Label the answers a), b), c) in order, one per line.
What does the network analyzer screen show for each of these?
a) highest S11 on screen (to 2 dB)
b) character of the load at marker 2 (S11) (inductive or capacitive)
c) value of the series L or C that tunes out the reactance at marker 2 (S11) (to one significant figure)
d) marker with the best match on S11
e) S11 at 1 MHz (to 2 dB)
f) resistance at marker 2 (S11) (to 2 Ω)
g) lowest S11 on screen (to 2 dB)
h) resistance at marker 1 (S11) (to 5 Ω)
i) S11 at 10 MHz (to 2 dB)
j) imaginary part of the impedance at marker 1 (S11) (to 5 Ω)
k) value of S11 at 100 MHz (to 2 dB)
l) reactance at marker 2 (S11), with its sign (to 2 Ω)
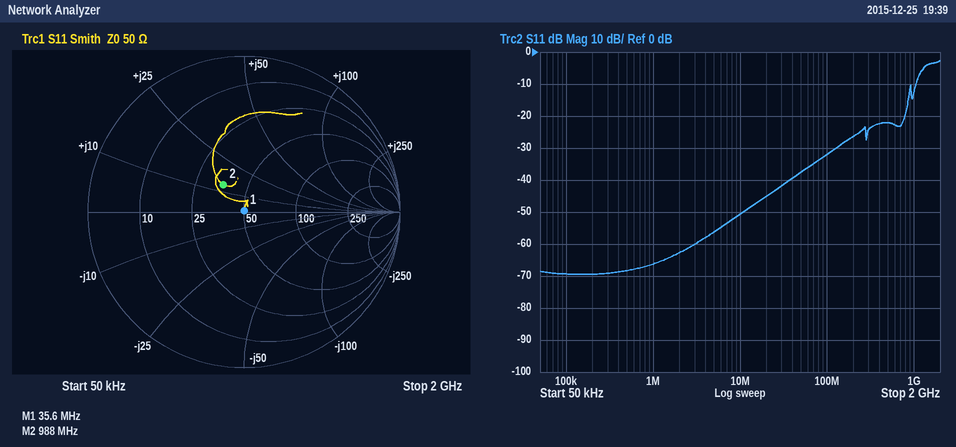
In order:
a) -2 dB
b) inductive
c) 10 pF
d) marker 1
e) -66 dB
f) 36 Ω
g) -70 dB
h) 50 Ω
i) -50 dB
j) 0 Ω
k) -32 dB
l) +14 Ω
